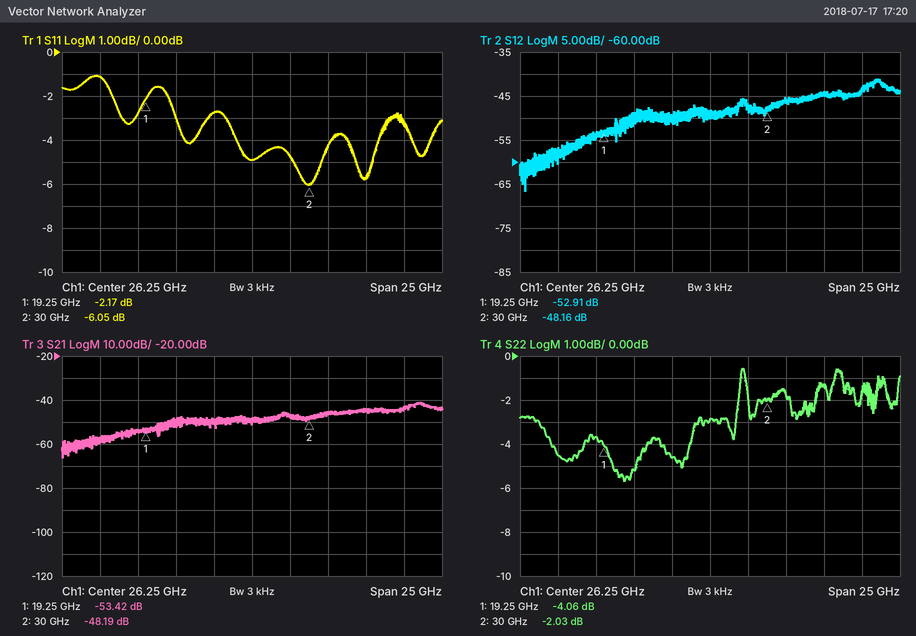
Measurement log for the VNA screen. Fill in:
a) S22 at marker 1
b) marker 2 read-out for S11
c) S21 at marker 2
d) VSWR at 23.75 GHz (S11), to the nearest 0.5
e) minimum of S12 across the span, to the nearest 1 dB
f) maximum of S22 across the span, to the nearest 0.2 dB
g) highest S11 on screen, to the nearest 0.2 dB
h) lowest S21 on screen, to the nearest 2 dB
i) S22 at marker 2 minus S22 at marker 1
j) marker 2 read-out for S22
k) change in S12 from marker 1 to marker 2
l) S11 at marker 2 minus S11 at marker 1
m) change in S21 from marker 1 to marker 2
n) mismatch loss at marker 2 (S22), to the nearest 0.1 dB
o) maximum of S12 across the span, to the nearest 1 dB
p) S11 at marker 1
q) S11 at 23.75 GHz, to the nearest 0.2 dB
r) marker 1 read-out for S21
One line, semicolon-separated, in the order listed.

-4.06 dB; -6.05 dB; -48.19 dB; 6.5; -67 dB; -0.6 dB; -1.0 dB; -66 dB; 2.03 dB; -2.03 dB; 4.75 dB; -3.88 dB; 5.23 dB; 4.3 dB; -41 dB; -2.17 dB; -2.8 dB; -53.42 dB
